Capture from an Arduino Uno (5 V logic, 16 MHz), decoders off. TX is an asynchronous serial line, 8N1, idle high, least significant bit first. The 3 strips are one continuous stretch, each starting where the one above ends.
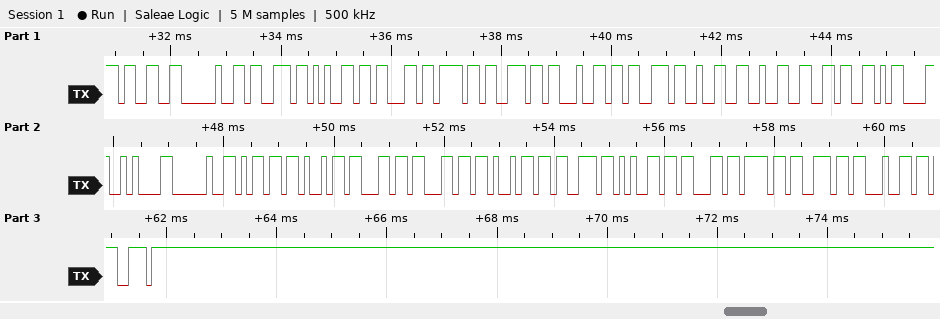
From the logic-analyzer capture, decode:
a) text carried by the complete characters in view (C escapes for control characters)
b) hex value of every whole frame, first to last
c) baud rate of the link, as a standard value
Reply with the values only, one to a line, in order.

"3 seconds226\r\n milliseconds"
0x33 0x20 0x73 0x65 0x63 0x6F 0x6E 0x64 0x73 0x32 0x32 0x36 0x0D 0x0A 0x20 0x6D 0x69 0x6C 0x6C 0x69 0x73 0x65 0x63 0x6F 0x6E 0x64 0x73
9600 baud
